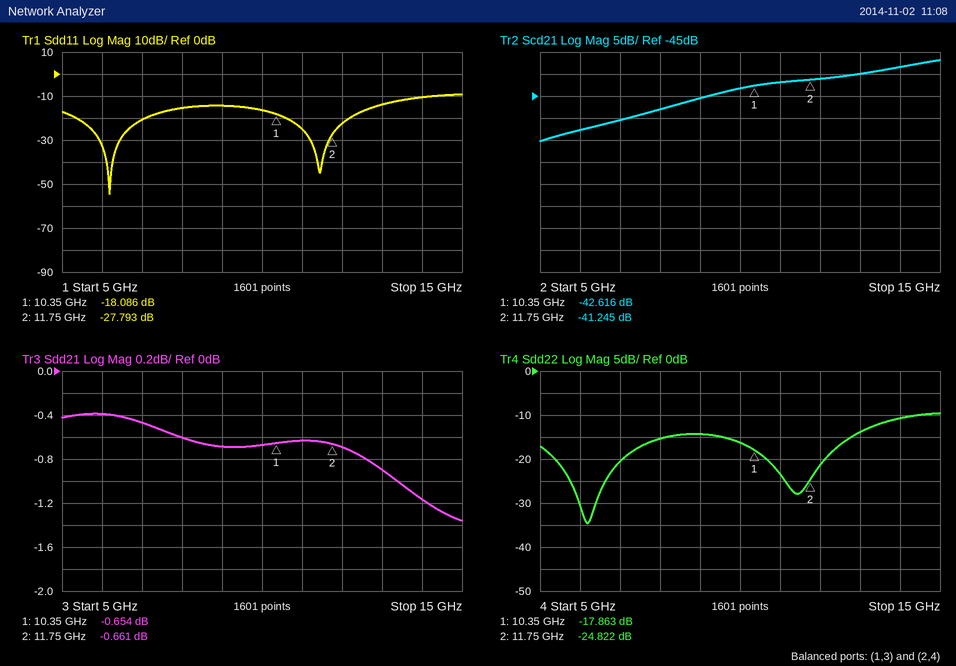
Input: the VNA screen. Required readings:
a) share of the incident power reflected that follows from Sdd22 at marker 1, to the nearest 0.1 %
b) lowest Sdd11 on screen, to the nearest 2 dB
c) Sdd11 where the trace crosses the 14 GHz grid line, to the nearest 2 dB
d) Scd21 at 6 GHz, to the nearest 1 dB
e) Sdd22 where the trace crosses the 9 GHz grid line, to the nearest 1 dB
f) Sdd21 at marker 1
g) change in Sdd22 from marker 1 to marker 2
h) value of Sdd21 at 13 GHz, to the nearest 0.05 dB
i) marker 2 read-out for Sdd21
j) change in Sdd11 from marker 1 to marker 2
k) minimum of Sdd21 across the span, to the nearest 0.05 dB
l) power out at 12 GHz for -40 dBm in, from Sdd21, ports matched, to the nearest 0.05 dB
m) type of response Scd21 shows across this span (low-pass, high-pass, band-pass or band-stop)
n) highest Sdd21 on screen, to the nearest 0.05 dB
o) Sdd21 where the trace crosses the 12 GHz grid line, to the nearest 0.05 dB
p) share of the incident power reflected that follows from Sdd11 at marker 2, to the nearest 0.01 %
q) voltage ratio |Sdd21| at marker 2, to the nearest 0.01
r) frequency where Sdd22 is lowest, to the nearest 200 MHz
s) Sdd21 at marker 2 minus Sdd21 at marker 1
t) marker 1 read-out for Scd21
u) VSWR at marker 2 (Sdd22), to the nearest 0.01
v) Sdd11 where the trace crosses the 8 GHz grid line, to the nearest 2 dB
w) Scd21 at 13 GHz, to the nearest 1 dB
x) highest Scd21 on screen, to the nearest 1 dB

1.6 %
-54 dB
-10 dB
-53 dB
-14 dB
-0.654 dB
-6.959 dB
-0.90 dB
-0.661 dB
-9.707 dB
-1.35 dB
-40.70 dBm
high-pass
-0.40 dB
-0.70 dB
0.17 %
0.93
6.2 GHz
-0.007 dB
-42.616 dB
1.12
-16 dB
-40 dB
-37 dB
